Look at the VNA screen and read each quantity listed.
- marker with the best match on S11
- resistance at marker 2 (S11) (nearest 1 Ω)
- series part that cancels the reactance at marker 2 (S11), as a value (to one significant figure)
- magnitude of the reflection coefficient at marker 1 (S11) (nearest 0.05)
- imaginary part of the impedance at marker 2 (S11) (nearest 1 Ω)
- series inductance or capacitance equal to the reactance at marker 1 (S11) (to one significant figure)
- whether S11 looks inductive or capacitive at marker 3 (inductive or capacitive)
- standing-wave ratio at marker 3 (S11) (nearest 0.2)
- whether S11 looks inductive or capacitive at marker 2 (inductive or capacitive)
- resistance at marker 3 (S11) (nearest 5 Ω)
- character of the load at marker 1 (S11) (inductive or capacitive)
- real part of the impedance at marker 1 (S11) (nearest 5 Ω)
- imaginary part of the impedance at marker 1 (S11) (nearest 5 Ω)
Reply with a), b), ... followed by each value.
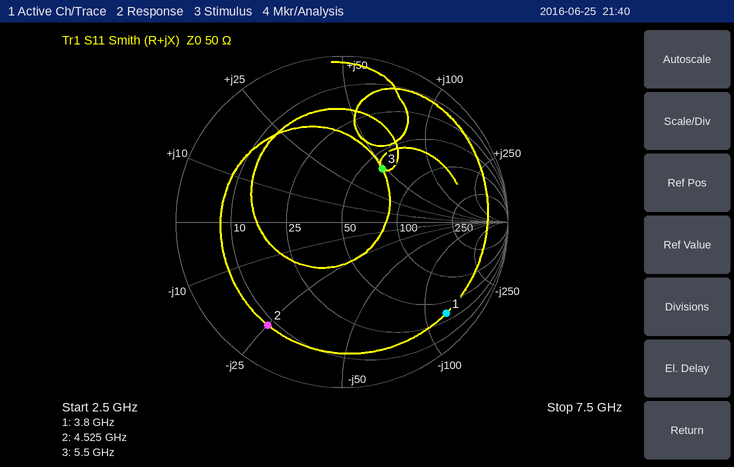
a) marker 3
b) 8 Ω
c) 900 pH
d) 0.85
e) -25 Ω
f) 300 fF
g) inductive
h) 2.4
i) capacitive
j) 60 Ω
k) capacitive
l) 35 Ω
m) -125 Ω
